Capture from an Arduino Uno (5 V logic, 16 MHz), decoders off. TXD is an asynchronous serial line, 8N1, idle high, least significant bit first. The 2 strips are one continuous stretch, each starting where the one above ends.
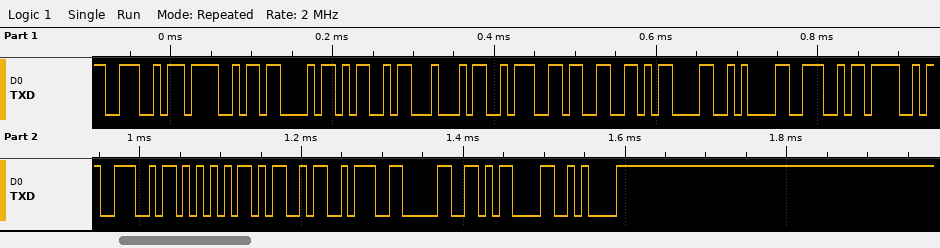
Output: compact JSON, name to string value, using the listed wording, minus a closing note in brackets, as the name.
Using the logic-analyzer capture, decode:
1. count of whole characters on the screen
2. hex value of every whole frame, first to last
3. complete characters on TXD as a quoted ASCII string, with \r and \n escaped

{"count of whole characters on the screen": "18", "hex value of every whole frame, first to last": "4E 4F 43 4D 44 3A 33 0D 0A 4E 4F 4E 55 4D 3A 30 0D 0A", "complete characters on TXD as a quoted ASCII string, with \\r and \\n escaped": "\"NOCMD:3\\r\\nNONUM:0\\r\\n\""}
